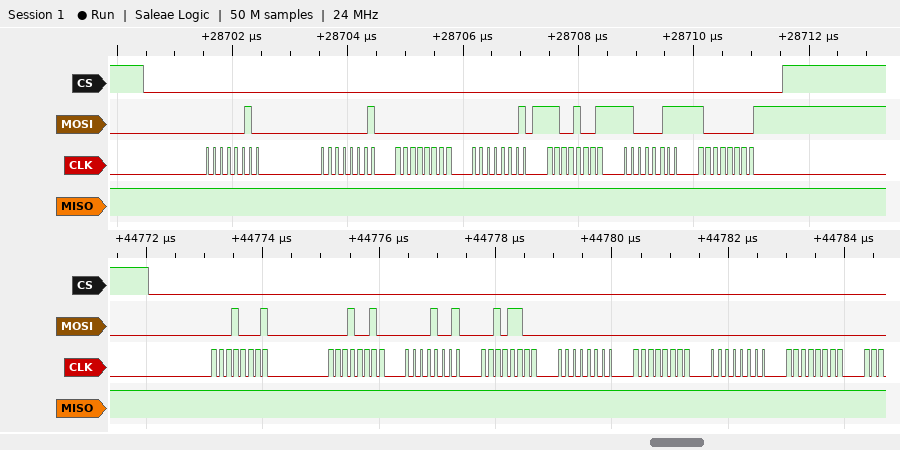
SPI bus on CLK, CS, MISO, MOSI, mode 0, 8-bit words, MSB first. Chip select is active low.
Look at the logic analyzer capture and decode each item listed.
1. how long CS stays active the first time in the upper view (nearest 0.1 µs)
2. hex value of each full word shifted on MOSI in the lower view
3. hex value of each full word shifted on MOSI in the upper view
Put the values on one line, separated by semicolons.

11.1 µs; 11, 12, 09, 2C, 00, 00, 00, 00; 02, 01, 00, 01, C9, C3, 80
